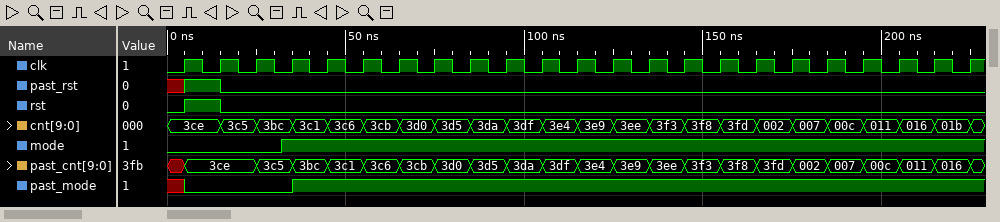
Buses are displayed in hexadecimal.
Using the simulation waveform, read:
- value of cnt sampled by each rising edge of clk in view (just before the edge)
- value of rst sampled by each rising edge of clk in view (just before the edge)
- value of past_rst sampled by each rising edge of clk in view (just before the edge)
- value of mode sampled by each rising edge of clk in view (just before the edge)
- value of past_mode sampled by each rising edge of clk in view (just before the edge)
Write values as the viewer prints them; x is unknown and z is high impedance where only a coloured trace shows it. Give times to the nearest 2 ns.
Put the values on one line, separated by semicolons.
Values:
3ce, 3ce, 3c5, 3bc, 3c1, 3c6, 3cb, 3d0, 3d5, 3da, 3df, 3e4, 3e9, 3ee, 3f3, 3f8, 3fd, 002, 007, 00c, 011, 016, 01b; 0 1 0 0 0 0 0 0 0 0 0 0 0 0 0 0 0 0 0 0 0 0 0; x 1 0 0 0 0 0 0 0 0 0 0 0 0 0 0 0 0 0 0 0 0 0; 0 0 0 1 1 1 1 1 1 1 1 1 1 1 1 1 1 1 1 1 1 1 1; x 0 0 0 1 1 1 1 1 1 1 1 1 1 1 1 1 1 1 1 1 1 1
